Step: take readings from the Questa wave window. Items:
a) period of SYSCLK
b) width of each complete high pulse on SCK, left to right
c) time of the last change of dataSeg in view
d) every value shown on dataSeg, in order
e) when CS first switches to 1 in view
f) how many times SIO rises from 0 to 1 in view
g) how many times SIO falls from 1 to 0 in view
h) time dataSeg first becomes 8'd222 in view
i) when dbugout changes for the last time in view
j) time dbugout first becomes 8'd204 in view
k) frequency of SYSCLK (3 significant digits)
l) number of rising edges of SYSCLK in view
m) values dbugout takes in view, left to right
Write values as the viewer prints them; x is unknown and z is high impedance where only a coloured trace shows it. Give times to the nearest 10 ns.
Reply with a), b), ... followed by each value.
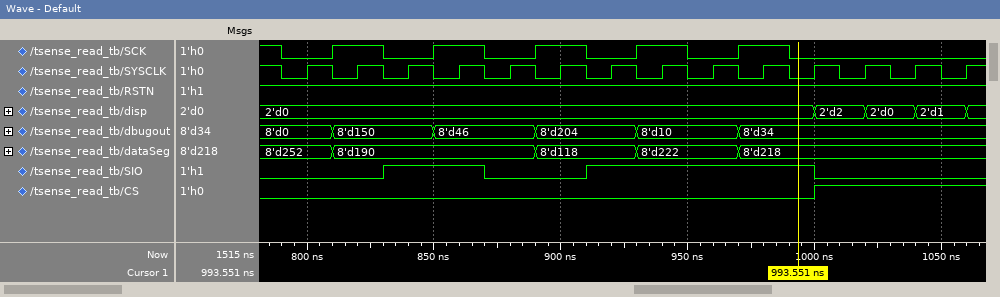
a) 20 ns
b) 20 ns, 20 ns, 20 ns, 20 ns, 20 ns
c) 970 ns
d) 8'd252, 8'd190, 8'd118, 8'd222, 8'd218
e) 1000 ns
f) 2
g) 2
h) 930 ns
i) 970 ns
j) 890 ns
k) 50.0 MHz
l) 14
m) 8'd0, 8'd150, 8'd46, 8'd204, 8'd10, 8'd34
